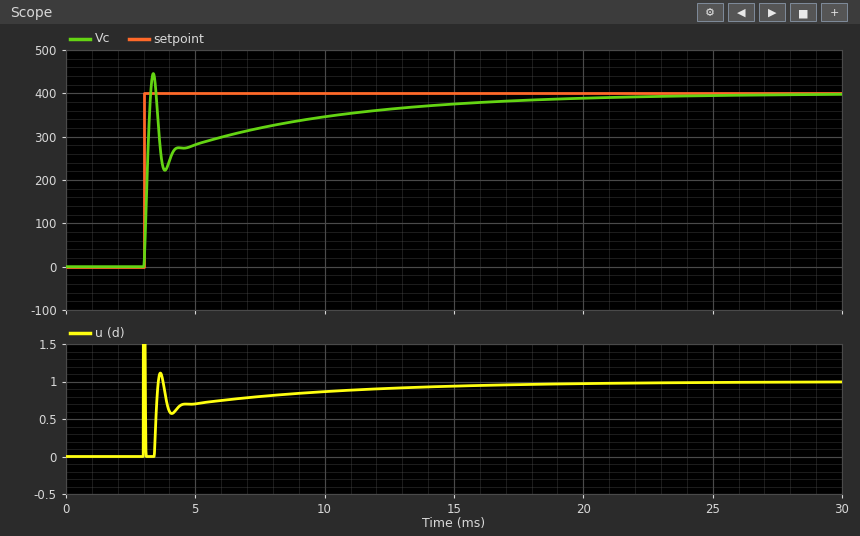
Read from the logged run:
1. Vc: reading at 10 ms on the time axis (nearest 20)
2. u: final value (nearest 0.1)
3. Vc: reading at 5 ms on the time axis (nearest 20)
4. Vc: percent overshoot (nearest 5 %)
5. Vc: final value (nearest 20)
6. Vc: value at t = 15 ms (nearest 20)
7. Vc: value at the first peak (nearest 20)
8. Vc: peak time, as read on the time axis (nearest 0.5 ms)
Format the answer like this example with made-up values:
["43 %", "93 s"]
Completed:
["340", "1.0", "280", "10 %", "400", "380", "440", "3.5 ms"]
